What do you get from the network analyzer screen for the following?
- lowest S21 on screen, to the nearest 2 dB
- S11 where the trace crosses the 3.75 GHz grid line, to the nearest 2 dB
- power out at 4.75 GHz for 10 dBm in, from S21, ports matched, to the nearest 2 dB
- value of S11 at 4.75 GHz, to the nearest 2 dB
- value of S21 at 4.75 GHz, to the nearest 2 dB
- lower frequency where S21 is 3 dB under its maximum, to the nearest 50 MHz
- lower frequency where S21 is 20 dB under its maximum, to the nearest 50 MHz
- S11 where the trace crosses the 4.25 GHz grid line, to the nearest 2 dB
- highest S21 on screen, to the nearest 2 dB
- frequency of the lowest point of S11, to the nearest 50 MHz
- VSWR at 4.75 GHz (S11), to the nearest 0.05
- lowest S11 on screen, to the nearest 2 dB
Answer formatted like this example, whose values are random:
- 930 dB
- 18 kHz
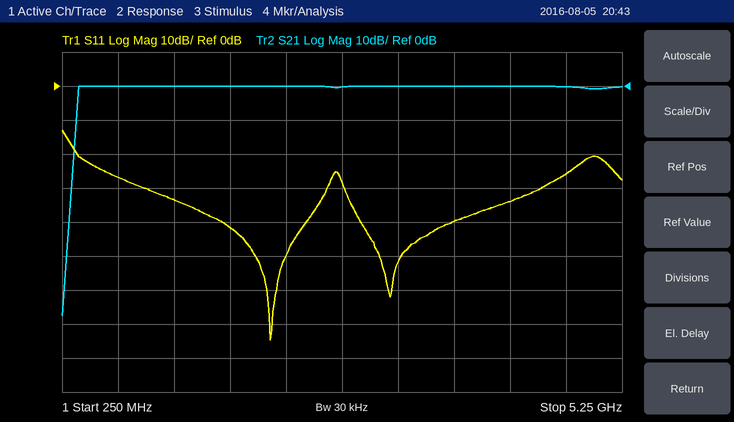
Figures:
- -68 dB
- -40 dB
- 10 dBm
- -26 dB
- 0 dB
- 400 MHz
- 350 MHz
- -34 dB
- 0 dB
- 2.10 GHz
- 1.10
- -74 dB
